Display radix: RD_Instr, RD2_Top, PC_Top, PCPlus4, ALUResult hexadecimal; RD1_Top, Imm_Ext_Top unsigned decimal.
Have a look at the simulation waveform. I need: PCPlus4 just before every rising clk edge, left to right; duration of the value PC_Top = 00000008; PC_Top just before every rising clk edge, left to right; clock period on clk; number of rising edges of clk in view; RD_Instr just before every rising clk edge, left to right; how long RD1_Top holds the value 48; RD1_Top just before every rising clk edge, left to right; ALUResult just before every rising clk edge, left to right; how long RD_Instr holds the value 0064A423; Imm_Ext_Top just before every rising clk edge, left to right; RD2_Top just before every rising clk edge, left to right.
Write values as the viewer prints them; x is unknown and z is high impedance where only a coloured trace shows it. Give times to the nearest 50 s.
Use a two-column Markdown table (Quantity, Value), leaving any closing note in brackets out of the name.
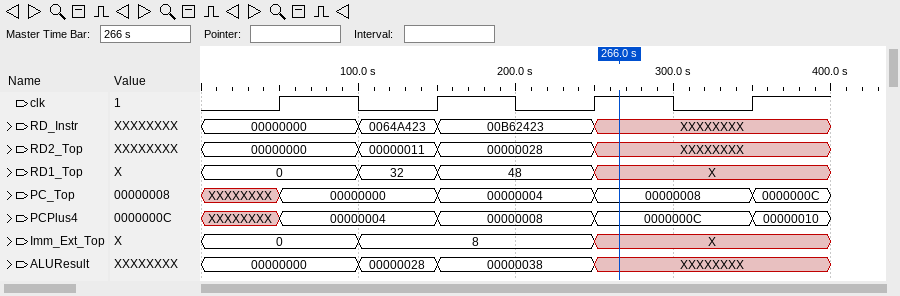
| Quantity | Value |
|---|---|
| PCPlus4 just before every rising clk edge, left to right | XXXXXXXX, 00000004, 00000008, 0000000C |
| duration of the value PC_Top = 00000008 | 100 s |
| PC_Top just before every rising clk edge, left to right | XXXXXXXX, 00000000, 00000004, 00000008 |
| clock period on clk | 100 s |
| number of rising edges of clk in view | 4 |
| RD_Instr just before every rising clk edge, left to right | 00000000, 0064A423, 00B62423, XXXXXXXX |
| how long RD1_Top holds the value 48 | 100 s |
| RD1_Top just before every rising clk edge, left to right | 0, 32, 48, X |
| ALUResult just before every rising clk edge, left to right | 00000000, 00000028, 00000038, XXXXXXXX |
| how long RD_Instr holds the value 0064A423 | 50 s |
| Imm_Ext_Top just before every rising clk edge, left to right | 0, 8, 8, X |
| RD2_Top just before every rising clk edge, left to right | 00000000, 00000011, 00000028, XXXXXXXX |
